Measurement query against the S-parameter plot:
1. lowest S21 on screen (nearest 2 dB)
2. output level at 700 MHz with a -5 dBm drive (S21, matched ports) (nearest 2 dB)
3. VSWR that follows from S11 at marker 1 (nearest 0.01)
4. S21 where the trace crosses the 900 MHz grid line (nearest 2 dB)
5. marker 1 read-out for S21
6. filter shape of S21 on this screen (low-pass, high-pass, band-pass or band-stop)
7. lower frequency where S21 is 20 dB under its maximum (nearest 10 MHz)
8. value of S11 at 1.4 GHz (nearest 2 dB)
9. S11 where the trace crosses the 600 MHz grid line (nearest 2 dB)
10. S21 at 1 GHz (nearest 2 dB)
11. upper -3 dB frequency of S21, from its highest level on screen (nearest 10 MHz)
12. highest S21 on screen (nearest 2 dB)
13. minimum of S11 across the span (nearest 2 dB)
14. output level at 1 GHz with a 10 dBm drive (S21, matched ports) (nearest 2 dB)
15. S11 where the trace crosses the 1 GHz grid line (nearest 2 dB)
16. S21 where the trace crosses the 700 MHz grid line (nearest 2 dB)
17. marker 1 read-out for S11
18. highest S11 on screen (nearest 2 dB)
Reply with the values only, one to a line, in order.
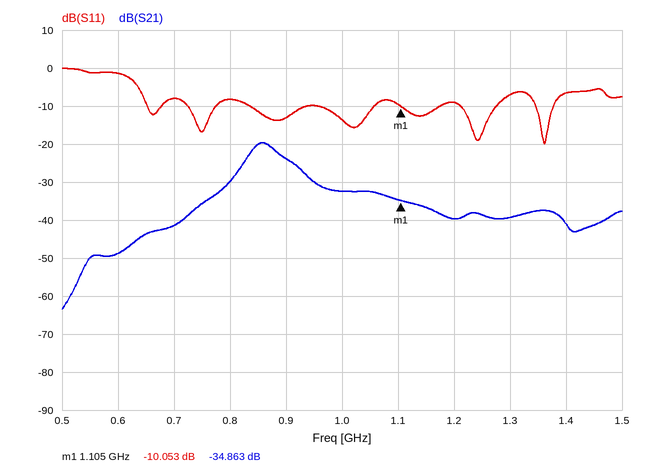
-64 dB
-46 dBm
1.92
-24 dB
-34.863 dB
band-pass
720 MHz
-6 dB
-2 dB
-32 dB
890 MHz
-20 dB
-20 dB
-22 dBm
-14 dB
-42 dB
-10.053 dB
0 dB
